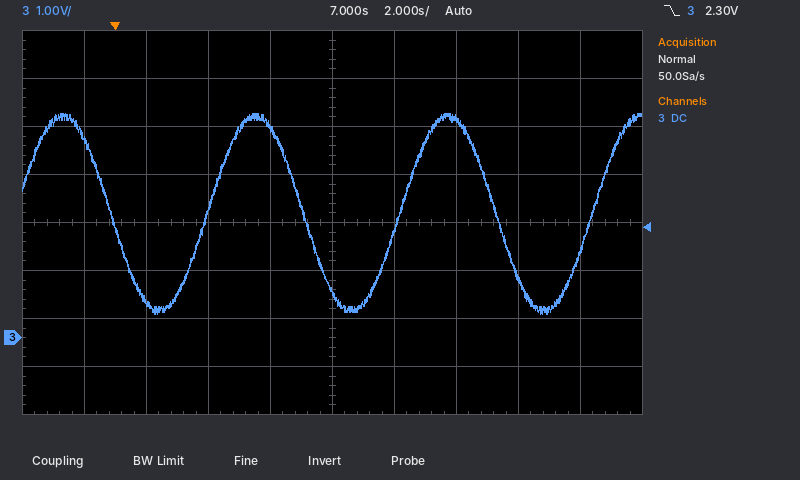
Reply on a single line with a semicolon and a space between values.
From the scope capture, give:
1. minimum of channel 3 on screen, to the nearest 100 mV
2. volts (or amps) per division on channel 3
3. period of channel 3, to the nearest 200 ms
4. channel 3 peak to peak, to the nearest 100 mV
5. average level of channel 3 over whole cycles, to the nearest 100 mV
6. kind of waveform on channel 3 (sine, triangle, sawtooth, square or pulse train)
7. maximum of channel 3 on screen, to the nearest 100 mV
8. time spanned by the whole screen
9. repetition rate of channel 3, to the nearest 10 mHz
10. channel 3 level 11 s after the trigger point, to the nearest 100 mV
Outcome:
500 mV; 1 V; 6.2 s; 4.2 V; 2.6 V; sine; 4.7 V; 20 s; 160 mHz; 4.5 V
